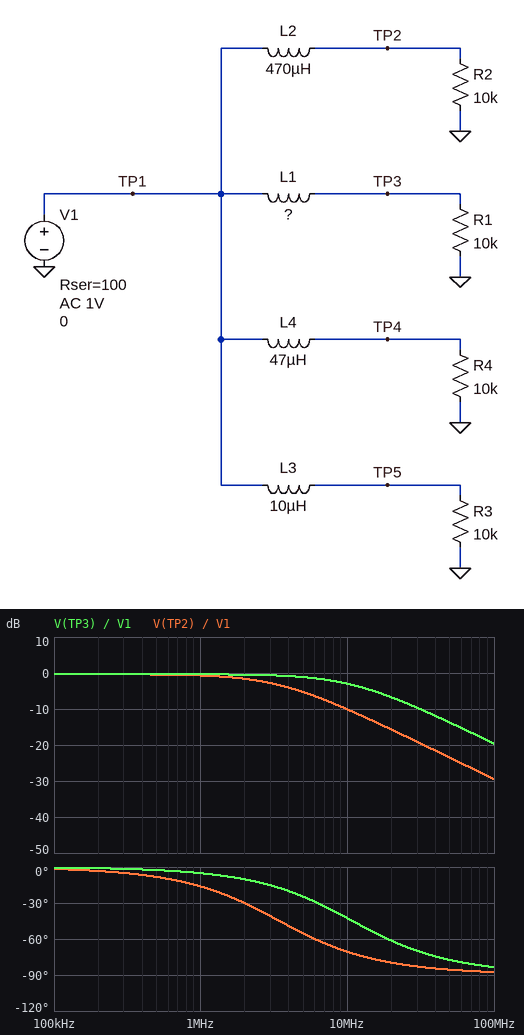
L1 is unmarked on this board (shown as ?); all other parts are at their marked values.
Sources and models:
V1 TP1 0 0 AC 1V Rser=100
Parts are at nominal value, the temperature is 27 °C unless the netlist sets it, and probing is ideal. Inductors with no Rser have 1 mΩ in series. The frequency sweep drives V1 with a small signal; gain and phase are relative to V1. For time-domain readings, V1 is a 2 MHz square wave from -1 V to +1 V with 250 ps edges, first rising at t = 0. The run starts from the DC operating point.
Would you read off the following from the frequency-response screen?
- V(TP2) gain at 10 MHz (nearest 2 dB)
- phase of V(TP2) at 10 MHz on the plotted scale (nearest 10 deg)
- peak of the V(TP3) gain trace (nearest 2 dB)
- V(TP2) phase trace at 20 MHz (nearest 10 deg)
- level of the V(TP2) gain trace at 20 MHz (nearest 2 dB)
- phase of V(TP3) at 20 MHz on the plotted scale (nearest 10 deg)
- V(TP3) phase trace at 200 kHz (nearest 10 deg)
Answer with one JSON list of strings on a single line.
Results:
["-10 dB", "-70 deg", "0 dB", "-80 deg", "-16 dB", "-60 deg", "0 deg"]
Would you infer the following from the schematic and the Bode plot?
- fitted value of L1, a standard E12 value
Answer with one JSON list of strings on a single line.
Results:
["150 µH"]
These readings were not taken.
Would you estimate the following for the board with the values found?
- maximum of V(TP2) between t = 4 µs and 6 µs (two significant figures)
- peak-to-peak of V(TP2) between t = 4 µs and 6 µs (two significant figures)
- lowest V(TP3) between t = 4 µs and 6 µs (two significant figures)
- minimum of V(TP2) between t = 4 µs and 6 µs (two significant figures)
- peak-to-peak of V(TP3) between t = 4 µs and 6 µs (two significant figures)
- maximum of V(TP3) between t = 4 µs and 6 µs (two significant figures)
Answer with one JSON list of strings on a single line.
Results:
["950 mV", "1.9 V", "-960 mV", "-950 mV", "1.9 V", "960 mV"]
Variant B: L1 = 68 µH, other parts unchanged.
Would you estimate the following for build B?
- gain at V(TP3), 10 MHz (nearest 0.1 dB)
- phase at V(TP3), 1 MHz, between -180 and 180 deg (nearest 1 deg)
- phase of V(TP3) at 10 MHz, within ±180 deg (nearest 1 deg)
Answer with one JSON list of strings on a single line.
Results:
["-1.0 dB", "-2 deg", "-23 deg"]
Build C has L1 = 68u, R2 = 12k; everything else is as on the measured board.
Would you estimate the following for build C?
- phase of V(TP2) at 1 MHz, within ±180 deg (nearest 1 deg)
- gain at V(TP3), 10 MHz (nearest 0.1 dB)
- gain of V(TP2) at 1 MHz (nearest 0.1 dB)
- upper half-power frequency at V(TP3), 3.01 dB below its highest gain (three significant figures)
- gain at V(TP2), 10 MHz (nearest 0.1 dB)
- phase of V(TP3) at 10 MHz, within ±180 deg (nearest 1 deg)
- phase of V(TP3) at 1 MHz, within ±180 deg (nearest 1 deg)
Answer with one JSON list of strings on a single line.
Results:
["-14 deg", "-1.0 dB", "-0.6 dB", "24.2 MHz", "-8.7 dB", "-23 deg", "-2 deg"]
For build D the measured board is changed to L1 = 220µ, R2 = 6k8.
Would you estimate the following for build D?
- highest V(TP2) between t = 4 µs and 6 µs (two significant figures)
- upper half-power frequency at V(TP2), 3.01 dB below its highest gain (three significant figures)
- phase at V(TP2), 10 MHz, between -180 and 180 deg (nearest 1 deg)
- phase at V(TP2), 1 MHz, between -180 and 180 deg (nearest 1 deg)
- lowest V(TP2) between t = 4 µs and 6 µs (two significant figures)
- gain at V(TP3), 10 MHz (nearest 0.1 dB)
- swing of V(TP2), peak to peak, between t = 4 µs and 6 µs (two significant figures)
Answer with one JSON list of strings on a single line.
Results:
["910 mV", "2.34 MHz", "-76 deg", "-23 deg", "-910 mV", "-4.8 dB", "1.8 V"]
